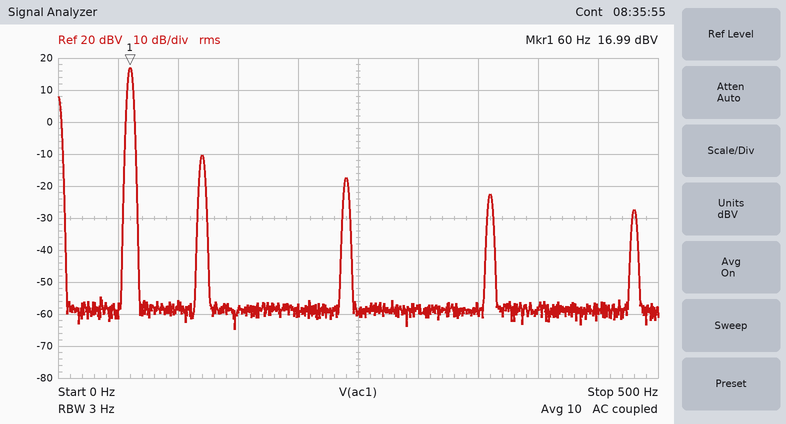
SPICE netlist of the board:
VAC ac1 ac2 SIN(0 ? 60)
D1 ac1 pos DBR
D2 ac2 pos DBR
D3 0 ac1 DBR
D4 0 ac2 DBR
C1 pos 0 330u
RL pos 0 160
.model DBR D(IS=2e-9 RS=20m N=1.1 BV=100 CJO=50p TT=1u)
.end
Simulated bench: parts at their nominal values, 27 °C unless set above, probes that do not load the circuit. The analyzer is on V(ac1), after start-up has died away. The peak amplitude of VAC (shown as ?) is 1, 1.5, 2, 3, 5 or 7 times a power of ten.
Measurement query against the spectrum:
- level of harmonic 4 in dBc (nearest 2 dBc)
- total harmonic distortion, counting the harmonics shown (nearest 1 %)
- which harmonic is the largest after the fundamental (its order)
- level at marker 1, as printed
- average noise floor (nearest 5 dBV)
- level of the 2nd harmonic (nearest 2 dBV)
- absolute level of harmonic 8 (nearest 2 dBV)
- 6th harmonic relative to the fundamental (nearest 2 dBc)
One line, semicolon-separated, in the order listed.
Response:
-34 dBc; 5 %; 2; 16.99 dBV; -60 dBV; -10 dBV; -28 dBV; -40 dBc
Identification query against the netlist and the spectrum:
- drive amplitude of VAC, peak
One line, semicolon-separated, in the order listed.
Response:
20 V
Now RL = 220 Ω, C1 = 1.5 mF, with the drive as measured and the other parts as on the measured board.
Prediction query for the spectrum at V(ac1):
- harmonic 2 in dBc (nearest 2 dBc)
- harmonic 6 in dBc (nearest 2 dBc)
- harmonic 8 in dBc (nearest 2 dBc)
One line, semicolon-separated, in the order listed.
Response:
-42 dBc; -52 dBc; -56 dBc
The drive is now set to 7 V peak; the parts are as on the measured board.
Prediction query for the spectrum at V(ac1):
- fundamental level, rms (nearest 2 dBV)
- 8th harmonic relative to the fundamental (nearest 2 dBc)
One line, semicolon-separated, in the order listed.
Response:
8 dBV; -46 dBc
